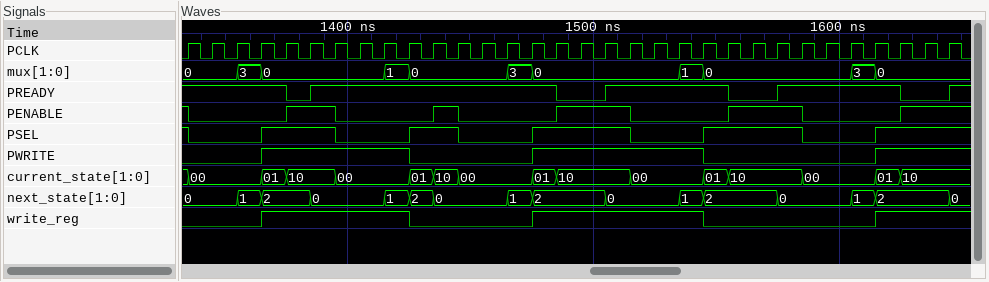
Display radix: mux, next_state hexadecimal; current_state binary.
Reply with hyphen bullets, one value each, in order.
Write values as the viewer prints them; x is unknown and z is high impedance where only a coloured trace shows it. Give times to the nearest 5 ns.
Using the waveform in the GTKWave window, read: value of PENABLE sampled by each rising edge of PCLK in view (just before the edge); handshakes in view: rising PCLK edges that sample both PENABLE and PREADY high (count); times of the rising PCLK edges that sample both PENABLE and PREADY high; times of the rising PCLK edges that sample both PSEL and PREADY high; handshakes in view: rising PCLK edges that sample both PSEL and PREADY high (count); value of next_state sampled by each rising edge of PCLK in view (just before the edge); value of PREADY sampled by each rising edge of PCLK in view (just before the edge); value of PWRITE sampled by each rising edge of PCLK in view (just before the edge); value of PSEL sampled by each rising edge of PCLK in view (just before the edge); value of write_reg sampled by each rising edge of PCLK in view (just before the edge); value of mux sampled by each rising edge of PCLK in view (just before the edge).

- 1 0 0 0 0 1 1 0 0 0 0 1 0 0 0 0 1 1 1 0 0 0 0 1 1 1 0 0 0 0 1 1
- 5
- 1335 ns, 1395 ns, 1445 ns, 1515 ns, 1585 ns
- 1335 ns, 1375 ns, 1395 ns, 1435 ns, 1445 ns, 1485 ns, 1515 ns, 1555 ns, 1585 ns, 1625 ns
- 10
- 0, 0, 0, 1, 2, 2, 0, 0, 0, 1, 2, 0, 0, 0, 1, 2, 2, 2, 0, 0, 0, 1, 2, 2, 2, 0, 0, 0, 1, 2, 2, 2
- 1 1 1 1 1 0 1 1 1 1 1 1 1 1 1 1 0 0 1 1 1 1 1 0 0 1 1 1 1 1 0 0
- 0 0 0 0 1 1 1 1 1 1 0 0 0 0 0 1 1 1 1 1 1 1 0 0 0 0 0 0 0 1 1 1
- 1 0 0 0 1 1 1 0 0 0 1 1 0 0 0 1 1 1 1 0 0 0 1 1 1 1 0 0 0 1 1 1
- 0 0 0 0 1 1 1 1 1 1 0 0 0 0 0 1 1 1 1 1 1 1 0 0 0 0 0 0 0 1 1 1
- 0, 0, 0, 3, 0, 0, 0, 0, 0, 1, 0, 0, 0, 0, 3, 0, 0, 0, 0, 0, 0, 1, 0, 0, 0, 0, 0, 0, 3, 0, 0, 0
